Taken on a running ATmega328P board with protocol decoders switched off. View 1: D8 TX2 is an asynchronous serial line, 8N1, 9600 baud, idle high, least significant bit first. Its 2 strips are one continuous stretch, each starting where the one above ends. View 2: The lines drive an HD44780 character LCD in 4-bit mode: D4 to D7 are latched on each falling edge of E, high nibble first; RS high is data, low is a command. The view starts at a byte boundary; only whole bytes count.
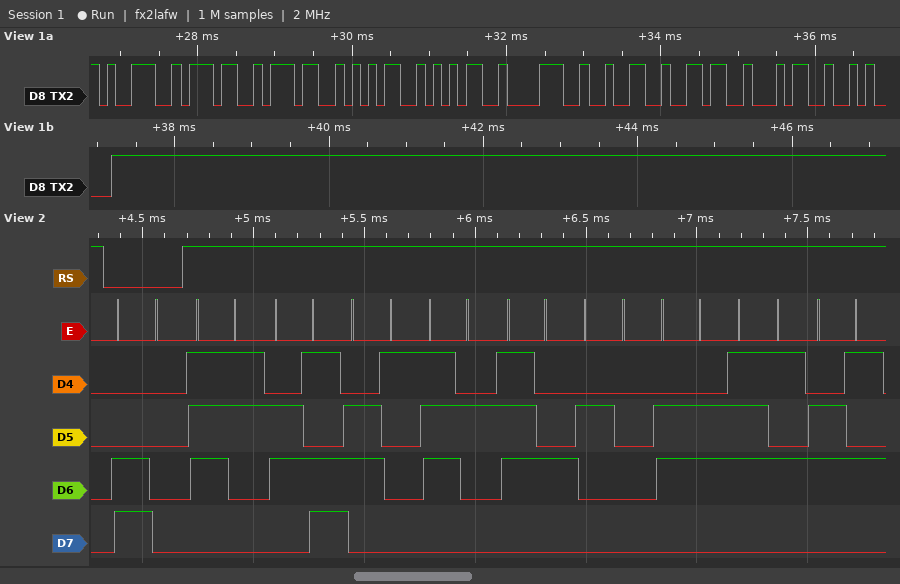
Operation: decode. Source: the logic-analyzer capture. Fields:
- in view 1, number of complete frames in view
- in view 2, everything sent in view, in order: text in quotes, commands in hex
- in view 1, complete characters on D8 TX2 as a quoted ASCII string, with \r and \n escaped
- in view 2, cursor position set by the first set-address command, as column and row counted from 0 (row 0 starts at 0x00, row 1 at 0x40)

10
0xC0 "smart fue"
"977558264\n"
column 0, row 1
